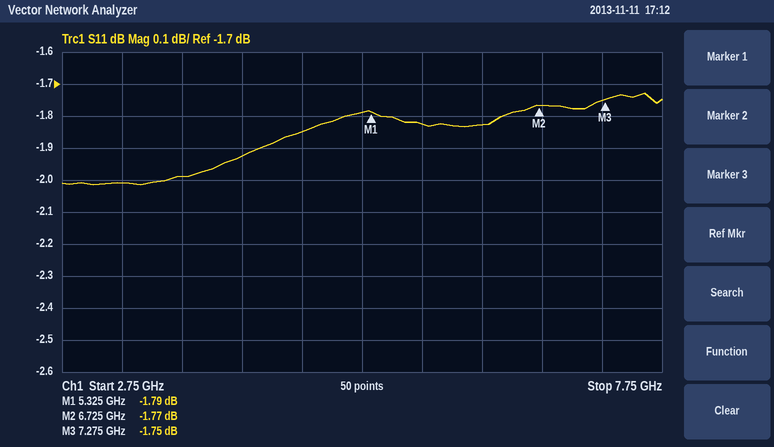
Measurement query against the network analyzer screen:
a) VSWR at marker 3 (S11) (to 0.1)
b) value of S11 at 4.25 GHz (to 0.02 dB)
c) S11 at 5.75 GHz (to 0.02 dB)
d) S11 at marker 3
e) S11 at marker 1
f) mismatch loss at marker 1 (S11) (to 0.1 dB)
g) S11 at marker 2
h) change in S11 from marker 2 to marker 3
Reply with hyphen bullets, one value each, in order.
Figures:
- 10.0
- -1.92 dB
- -1.82 dB
- -1.75 dB
- -1.79 dB
- 4.7 dB
- -1.77 dB
- 0.02 dB
